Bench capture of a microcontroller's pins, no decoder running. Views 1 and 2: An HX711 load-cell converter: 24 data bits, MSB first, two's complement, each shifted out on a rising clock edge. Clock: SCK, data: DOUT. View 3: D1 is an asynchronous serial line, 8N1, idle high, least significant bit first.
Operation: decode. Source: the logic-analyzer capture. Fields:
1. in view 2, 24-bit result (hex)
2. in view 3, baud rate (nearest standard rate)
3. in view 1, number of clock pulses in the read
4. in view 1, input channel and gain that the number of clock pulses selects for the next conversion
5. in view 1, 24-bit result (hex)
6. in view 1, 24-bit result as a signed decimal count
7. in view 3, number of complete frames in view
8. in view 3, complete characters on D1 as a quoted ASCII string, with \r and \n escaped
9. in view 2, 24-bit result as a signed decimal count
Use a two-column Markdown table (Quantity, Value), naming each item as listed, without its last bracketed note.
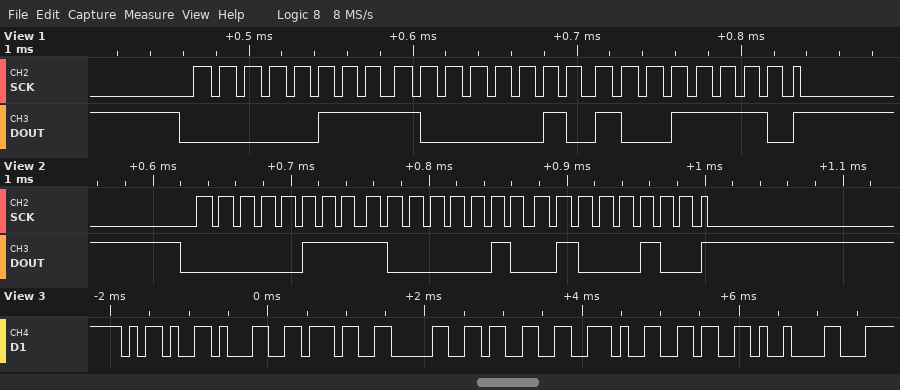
| Quantity | Value |
|---|---|
| in view 2, 24-bit result | 0x078244 |
| in view 3, baud rate | 9600 baud |
| in view 1, number of clock pulses in the read | 25 |
| in view 1, input channel and gain that the number of clock pulses selects for the next conversion | channel A, gain 128 |
| in view 1, 24-bit result | 0x07829E |
| in view 1, 24-bit result as a signed decimal count | 492190 |
| in view 3, number of complete frames in view | 8 |
| in view 3, complete characters on D1 as a quoted ASCII string, with \r and \n escaped | "-1703.6\t" |
| in view 2, 24-bit result as a signed decimal count | 492100 |
